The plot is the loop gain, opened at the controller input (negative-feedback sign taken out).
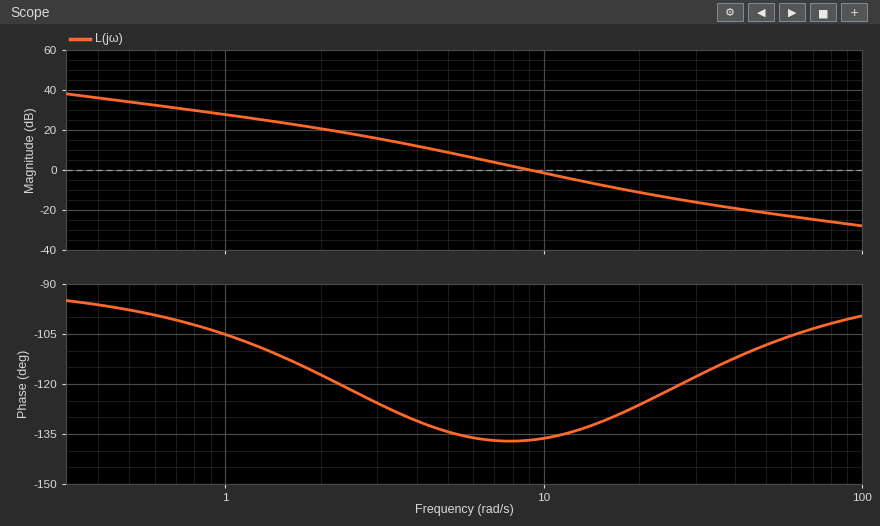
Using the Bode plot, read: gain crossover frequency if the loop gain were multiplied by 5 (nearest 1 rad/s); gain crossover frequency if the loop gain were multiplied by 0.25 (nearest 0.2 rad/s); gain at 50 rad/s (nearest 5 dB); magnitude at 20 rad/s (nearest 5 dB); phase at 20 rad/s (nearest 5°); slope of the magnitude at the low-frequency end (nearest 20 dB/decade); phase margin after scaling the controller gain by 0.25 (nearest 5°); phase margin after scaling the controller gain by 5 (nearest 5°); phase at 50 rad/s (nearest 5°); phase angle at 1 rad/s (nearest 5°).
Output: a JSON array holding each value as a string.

["25 rad/s", "4.0 rad/s", "-20 dB", "-10 dB", "-125°", "-20 dB/decade", "50°", "60°", "-110°", "-105°"]
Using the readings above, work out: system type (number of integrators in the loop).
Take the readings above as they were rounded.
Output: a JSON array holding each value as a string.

["1"]
